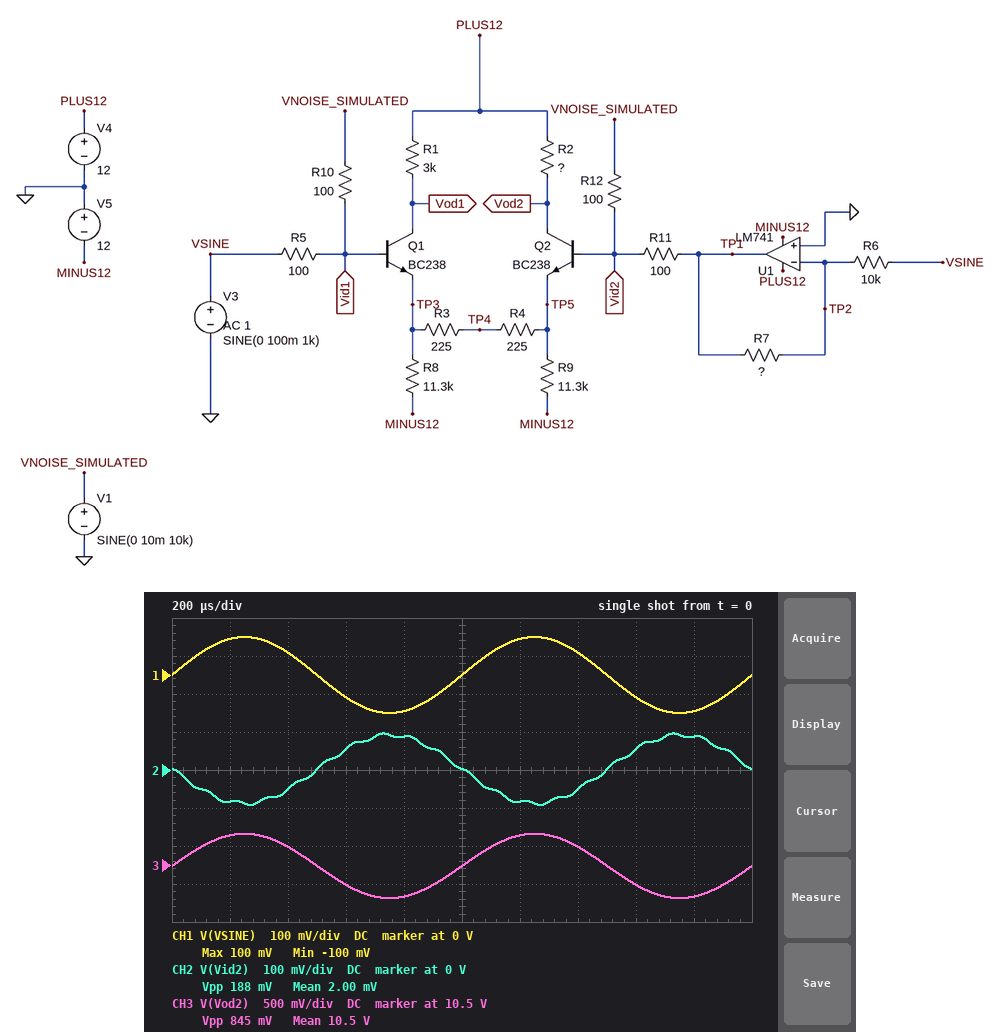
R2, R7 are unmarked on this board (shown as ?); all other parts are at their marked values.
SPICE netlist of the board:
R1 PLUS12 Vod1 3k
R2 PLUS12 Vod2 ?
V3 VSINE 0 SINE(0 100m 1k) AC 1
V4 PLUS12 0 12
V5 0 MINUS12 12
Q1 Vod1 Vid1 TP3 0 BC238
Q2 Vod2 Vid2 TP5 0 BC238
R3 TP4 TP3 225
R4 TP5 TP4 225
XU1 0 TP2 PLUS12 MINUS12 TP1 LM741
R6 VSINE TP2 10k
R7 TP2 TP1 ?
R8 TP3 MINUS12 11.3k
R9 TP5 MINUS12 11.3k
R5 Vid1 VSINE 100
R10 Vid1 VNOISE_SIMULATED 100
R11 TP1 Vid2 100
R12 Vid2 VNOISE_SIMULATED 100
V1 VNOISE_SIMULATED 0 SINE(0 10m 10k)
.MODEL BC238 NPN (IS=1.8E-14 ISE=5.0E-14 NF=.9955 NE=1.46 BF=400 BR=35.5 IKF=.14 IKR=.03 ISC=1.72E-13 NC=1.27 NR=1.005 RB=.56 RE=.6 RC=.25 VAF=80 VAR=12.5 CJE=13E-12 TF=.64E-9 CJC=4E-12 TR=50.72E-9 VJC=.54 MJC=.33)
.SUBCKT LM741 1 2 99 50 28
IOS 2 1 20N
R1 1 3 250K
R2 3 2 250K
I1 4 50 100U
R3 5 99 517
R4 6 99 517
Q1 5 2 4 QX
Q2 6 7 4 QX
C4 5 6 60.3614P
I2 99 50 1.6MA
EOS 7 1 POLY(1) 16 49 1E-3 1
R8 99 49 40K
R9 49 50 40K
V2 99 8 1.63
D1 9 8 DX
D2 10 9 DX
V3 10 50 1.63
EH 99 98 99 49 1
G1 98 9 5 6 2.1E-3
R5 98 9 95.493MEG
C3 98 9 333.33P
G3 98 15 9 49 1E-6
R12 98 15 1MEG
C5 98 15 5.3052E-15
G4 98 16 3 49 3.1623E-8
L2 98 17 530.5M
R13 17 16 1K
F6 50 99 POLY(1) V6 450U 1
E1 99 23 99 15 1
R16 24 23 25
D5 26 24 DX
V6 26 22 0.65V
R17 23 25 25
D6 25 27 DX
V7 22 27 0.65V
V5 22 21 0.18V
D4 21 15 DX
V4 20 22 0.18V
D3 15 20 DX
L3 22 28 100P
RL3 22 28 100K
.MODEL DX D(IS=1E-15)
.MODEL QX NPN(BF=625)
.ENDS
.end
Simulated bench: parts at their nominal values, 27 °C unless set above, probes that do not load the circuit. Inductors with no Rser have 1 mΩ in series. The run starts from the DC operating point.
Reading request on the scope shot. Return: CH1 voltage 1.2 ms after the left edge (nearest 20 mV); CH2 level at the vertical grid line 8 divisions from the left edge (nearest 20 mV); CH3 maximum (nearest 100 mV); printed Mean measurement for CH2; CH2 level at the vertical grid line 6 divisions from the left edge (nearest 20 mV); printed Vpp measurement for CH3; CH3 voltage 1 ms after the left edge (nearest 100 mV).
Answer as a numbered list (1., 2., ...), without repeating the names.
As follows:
1. 100 mV
2. 60 mV
3. 10.9 V
4. 2.00 mV
5. -80 mV
6. 845 mV
7. 10.5 V
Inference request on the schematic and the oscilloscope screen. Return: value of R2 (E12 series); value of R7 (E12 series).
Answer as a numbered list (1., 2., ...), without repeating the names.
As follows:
1. 1.5 kΩ
2. 18 kΩ
